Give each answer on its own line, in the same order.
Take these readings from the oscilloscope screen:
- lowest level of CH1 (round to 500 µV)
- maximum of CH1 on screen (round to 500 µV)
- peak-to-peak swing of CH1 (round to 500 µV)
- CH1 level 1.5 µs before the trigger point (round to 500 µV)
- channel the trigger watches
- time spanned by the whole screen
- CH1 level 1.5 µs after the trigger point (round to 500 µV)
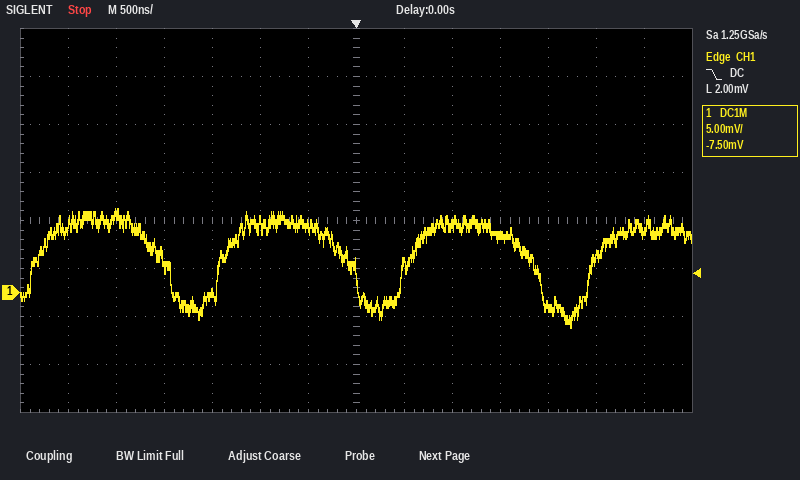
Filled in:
-3.5 mV
9.0 mV
12.5 mV
0.0 mV
CH1
7 µs
6.0 mV
